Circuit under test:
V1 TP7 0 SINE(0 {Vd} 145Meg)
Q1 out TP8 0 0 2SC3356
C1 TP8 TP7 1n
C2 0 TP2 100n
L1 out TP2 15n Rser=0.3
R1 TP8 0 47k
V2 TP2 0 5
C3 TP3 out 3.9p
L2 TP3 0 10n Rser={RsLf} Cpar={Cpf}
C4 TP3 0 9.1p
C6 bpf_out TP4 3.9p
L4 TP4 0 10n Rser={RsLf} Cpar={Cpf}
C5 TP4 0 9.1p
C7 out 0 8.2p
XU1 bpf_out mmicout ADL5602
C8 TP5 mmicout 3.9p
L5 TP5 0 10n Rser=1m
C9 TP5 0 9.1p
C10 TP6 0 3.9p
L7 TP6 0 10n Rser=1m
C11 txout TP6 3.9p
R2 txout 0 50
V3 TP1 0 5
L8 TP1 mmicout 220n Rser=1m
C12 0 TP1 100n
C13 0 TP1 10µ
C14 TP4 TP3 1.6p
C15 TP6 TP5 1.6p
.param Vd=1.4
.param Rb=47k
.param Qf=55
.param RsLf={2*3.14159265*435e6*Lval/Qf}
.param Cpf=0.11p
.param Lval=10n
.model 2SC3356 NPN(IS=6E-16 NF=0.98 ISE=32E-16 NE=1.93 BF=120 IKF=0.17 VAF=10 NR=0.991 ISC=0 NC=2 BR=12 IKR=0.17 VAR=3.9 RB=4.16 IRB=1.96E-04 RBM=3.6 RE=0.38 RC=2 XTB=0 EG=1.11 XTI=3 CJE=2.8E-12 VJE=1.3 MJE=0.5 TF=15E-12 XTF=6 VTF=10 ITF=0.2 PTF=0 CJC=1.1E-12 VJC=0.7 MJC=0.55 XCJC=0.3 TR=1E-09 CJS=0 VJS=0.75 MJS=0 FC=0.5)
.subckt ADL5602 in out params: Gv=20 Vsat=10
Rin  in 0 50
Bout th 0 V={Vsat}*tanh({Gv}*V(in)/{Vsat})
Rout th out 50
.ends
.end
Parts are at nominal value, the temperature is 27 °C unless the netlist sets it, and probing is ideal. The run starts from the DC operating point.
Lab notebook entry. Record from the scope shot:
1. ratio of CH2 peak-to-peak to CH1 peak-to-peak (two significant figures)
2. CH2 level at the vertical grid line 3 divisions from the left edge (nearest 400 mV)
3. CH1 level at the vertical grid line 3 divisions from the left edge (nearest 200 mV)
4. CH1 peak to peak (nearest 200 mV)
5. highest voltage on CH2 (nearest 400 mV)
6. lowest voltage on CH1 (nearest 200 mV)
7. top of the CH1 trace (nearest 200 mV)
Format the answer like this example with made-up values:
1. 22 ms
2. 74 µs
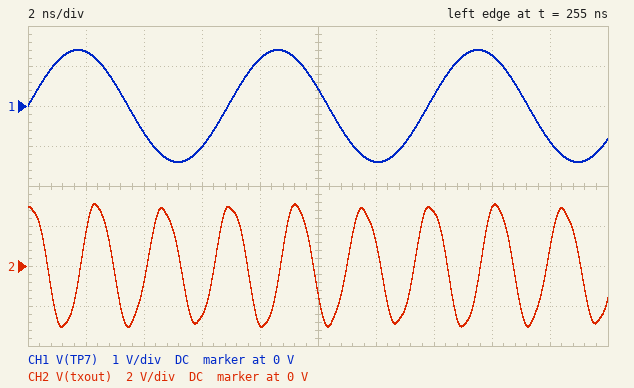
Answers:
1. 2.2
2. -2.4 V
3. -1.0 V
4. 2.8 V
5. 3.2 V
6. -1.4 V
7. 1.4 V
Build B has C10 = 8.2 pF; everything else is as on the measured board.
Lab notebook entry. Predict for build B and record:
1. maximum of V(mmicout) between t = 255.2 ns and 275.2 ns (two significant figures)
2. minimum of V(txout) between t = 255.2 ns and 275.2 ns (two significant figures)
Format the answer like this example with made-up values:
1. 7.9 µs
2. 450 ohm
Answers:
1. 13 V
2. -5.8 V
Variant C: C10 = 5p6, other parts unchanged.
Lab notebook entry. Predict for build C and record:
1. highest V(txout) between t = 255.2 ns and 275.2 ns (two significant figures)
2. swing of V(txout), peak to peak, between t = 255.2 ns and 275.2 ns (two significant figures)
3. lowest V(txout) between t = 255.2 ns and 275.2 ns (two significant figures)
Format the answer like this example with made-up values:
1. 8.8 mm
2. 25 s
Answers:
1. 3.9 V
2. 7.8 V
3. -3.9 V
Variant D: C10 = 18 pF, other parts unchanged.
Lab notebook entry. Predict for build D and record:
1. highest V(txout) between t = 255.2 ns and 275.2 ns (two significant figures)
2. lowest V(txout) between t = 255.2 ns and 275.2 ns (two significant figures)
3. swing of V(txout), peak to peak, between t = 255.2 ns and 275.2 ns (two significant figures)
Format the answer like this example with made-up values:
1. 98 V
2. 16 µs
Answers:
1. 1.9 V
2. -1.9 V
3. 3.8 V
